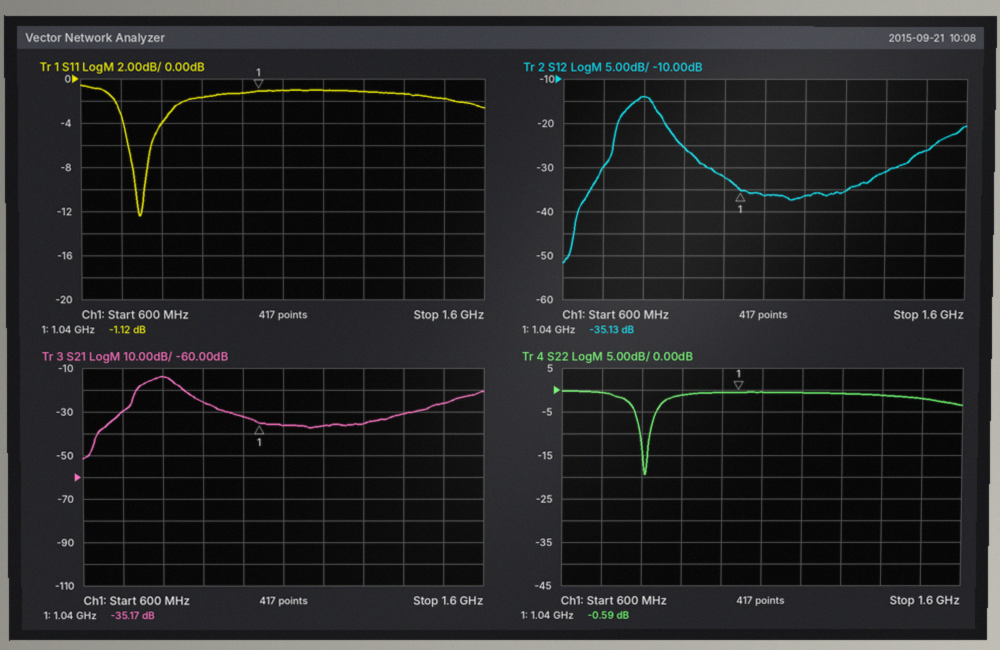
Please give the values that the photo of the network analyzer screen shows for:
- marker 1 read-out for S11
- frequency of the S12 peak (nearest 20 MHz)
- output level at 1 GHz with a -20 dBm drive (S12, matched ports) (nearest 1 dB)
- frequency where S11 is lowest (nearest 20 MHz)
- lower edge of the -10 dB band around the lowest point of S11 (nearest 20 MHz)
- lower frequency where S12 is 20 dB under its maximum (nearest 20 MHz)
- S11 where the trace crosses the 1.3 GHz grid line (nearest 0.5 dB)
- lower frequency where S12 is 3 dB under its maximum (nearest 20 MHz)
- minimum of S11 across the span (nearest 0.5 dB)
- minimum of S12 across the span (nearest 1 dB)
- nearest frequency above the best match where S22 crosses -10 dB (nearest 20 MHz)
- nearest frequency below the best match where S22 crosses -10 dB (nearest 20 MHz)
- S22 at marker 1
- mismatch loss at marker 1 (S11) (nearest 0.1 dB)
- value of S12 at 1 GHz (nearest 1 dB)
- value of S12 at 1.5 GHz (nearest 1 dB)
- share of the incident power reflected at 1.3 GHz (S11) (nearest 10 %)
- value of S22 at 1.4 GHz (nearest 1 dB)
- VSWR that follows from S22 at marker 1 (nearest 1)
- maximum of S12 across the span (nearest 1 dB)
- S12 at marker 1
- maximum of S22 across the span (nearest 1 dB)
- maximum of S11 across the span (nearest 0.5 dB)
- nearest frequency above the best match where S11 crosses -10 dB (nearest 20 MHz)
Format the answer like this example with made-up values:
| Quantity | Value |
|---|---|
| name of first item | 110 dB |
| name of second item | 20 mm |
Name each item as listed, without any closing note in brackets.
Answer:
| Quantity | Value |
|---|---|
| marker 1 read-out for S11 | -1.12 dB |
| frequency of the S12 peak | 800 MHz |
| output level at 1 GHz with a -20 dBm drive (S12, matched ports) | -52 dBm |
| frequency where S11 is lowest | 740 MHz |
| lower edge of the -10 dB band around the lowest point of S11 | 740 MHz |
| lower frequency where S12 is 20 dB under its maximum | 680 MHz |
| S11 where the trace crosses the 1.3 GHz grid line | -1.0 dB |
| lower frequency where S12 is 3 dB under its maximum | 760 MHz |
| minimum of S11 across the span | -12.5 dB |
| minimum of S12 across the span | -52 dB |
| nearest frequency above the best match where S22 crosses -10 dB | 820 MHz |
| nearest frequency below the best match where S22 crosses -10 dB | 800 MHz |
| S22 at marker 1 | -0.59 dB |
| mismatch loss at marker 1 (S11) | 6.4 dB |
| value of S12 at 1 GHz | -32 dB |
| value of S12 at 1.5 GHz | -26 dB |
| share of the incident power reflected at 1.3 GHz (S11) | 80 % |
| value of S22 at 1.4 GHz | -1 dB |
| VSWR that follows from S22 at marker 1 | 29 |
| maximum of S12 across the span | -14 dB |
| S12 at marker 1 | -35.13 dB |
| maximum of S22 across the span | 0 dB |
| maximum of S11 across the span | -0.5 dB |
| nearest frequency above the best match where S11 crosses -10 dB | 760 MHz |
